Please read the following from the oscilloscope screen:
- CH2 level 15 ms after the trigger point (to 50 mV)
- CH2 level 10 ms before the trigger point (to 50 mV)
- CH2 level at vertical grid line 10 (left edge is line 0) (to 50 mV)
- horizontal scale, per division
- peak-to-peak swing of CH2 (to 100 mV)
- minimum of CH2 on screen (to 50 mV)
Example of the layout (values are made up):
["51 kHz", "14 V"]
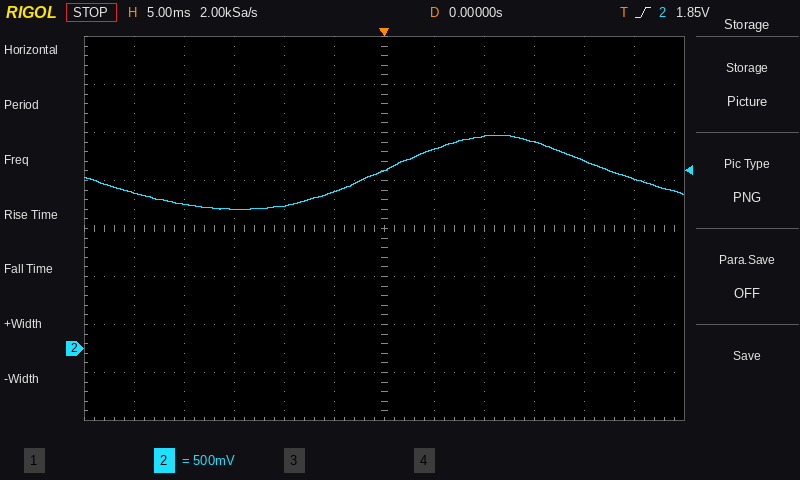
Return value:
["2.15 V", "1.50 V", "1.95 V", "5 ms", "800 mV", "1.45 V"]
